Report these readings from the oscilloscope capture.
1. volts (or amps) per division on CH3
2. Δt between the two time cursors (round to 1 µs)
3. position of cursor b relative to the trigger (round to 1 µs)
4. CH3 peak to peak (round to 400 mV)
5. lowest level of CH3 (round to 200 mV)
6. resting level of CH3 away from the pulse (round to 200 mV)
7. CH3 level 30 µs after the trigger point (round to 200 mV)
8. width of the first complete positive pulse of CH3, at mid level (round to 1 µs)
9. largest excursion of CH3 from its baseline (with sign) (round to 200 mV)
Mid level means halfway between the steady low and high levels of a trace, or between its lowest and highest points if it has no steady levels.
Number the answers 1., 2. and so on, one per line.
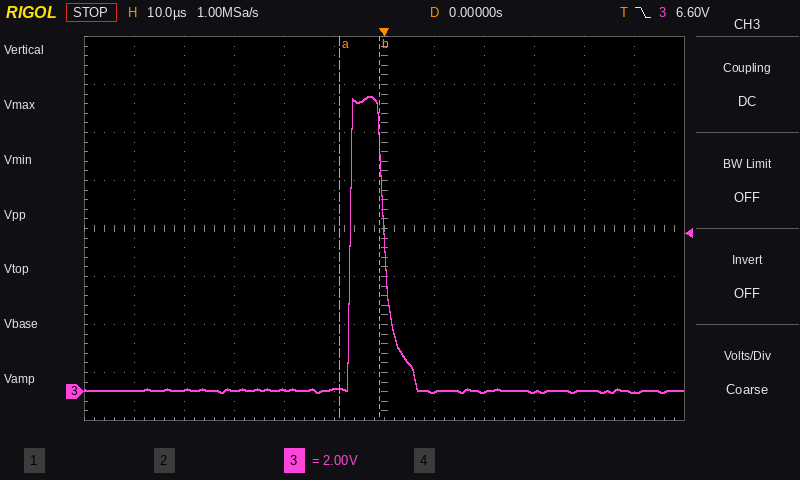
1. 2 V
2. 8 µs
3. -1 µs
4. 12.4 V
5. 0.0 V
6. 0.0 V
7. 0.0 V
8. 7 µs
9. +12.2 V
